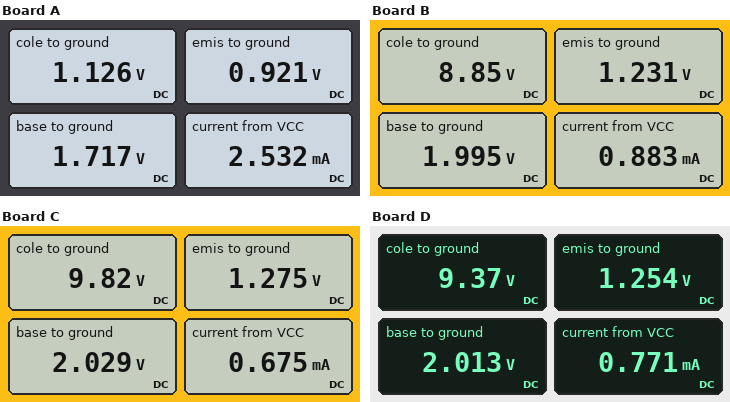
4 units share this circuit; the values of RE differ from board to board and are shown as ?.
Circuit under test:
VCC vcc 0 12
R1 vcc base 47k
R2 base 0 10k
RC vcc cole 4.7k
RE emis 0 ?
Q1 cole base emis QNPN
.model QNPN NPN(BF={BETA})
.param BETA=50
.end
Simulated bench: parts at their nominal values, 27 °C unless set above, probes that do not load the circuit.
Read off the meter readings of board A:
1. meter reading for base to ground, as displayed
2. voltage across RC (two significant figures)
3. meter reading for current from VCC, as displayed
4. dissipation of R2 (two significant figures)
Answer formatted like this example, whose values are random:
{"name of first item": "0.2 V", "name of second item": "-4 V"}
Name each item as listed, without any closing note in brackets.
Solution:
{"meter reading for base to ground, as displayed": "1.717 V", "voltage across RC": "11 V", "meter reading for current from VCC, as displayed": "2.532 mA", "dissipation of R2": "290 µW"}
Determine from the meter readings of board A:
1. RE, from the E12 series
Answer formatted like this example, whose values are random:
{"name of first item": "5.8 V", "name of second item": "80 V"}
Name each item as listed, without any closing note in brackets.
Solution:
{"RE, from the E12 series": "390 Ω"}
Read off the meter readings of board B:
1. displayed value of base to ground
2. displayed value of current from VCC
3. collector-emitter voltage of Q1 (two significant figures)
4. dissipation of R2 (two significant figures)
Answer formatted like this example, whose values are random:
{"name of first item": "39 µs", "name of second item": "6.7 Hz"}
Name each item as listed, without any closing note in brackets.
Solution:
{"displayed value of base to ground": "1.995 V", "displayed value of current from VCC": "0.883 mA", "collector-emitter voltage of Q1": "7.6 V", "dissipation of R2": "400 µW"}
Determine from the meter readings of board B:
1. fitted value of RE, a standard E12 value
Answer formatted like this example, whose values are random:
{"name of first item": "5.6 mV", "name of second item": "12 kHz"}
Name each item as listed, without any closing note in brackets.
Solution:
{"fitted value of RE, a standard E12 value": "1.8 kΩ"}
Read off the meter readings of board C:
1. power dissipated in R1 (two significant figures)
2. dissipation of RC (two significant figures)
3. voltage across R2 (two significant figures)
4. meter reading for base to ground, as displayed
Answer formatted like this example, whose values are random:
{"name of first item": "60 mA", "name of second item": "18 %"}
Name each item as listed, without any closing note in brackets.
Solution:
{"power dissipated in R1": "2.1 mW", "dissipation of RC": "1.0 mW", "voltage across R2": "2.0 V", "meter reading for base to ground, as displayed": "2.029 V"}
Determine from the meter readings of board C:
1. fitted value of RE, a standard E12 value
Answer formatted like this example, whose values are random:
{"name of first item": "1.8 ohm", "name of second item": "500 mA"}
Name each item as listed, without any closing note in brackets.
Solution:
{"fitted value of RE, a standard E12 value": "2.7 kΩ"}
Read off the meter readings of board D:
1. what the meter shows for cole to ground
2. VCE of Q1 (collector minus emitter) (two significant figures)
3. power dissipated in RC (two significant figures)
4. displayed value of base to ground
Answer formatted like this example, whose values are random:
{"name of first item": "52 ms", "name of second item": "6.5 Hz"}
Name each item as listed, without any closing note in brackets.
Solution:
{"what the meter shows for cole to ground": "9.37 V", "VCE of Q1 (collector minus emitter)": "8.1 V", "power dissipated in RC": "1.5 mW", "displayed value of base to ground": "2.013 V"}
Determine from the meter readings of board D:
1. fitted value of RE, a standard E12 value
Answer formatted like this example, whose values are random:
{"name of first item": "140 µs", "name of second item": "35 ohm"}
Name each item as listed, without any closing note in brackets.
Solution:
{"fitted value of RE, a standard E12 value": "2.2 kΩ"}
